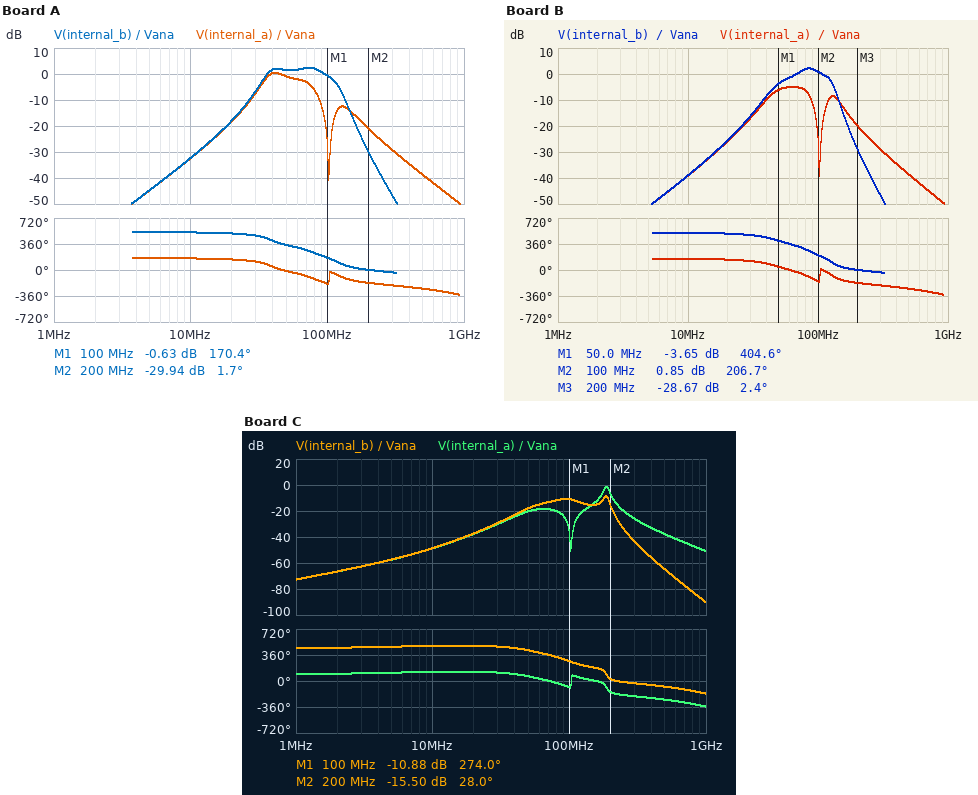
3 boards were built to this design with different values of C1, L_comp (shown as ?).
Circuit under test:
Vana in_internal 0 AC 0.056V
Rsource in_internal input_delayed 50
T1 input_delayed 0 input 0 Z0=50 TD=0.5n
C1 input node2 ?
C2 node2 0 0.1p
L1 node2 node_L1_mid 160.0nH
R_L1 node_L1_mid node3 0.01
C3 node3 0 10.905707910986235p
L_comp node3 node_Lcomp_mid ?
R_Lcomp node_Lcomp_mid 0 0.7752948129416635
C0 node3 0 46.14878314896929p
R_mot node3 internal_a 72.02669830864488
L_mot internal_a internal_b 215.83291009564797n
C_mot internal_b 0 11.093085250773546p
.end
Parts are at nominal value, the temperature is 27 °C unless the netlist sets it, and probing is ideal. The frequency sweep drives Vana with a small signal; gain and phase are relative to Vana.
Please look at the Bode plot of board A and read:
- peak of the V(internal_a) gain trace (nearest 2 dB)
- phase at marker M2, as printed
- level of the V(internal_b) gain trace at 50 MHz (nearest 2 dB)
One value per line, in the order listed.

0 dB
1.7 deg
2 dB
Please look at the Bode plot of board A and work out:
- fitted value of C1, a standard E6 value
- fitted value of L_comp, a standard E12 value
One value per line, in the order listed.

47 pF
120 nH
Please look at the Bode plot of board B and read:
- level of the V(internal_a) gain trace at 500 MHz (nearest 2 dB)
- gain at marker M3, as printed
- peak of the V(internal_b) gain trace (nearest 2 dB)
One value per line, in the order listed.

-38 dB
-28.67 dB
2 dB
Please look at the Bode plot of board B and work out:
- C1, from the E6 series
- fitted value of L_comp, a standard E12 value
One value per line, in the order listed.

47 pF
56 nH
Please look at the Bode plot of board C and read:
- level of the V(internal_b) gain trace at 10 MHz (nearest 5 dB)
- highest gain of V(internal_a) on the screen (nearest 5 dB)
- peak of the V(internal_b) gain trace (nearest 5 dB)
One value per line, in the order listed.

-50 dB
0 dB
-10 dB
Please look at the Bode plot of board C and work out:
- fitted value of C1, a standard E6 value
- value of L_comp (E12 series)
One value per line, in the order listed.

47 pF
15 nH
